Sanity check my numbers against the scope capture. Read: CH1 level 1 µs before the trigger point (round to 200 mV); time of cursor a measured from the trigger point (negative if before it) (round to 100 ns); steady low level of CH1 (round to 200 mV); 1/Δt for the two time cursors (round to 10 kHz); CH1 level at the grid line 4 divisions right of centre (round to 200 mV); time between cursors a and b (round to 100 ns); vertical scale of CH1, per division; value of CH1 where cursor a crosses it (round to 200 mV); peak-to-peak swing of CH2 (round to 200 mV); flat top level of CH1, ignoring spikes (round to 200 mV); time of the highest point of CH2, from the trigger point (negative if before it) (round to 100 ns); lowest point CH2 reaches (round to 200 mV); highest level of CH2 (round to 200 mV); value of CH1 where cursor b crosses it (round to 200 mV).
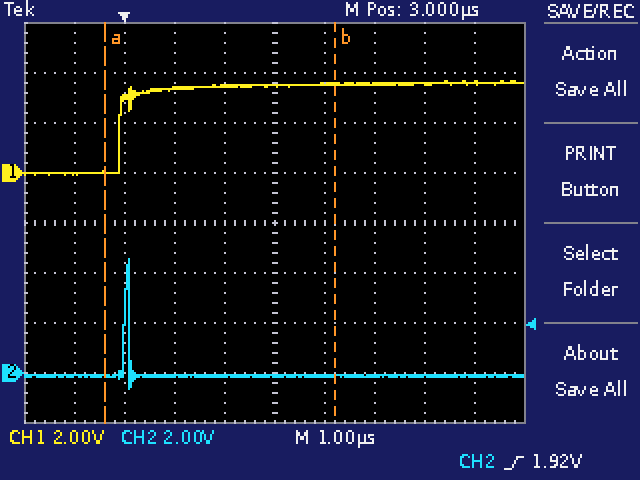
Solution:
0.0 V
-400 ns
0.0 V
220 kHz
3.6 V
4.6 µs
2 V
0.0 V
5.2 V
3.6 V
+100 ns
-600 mV
4.6 V
3.6 V
